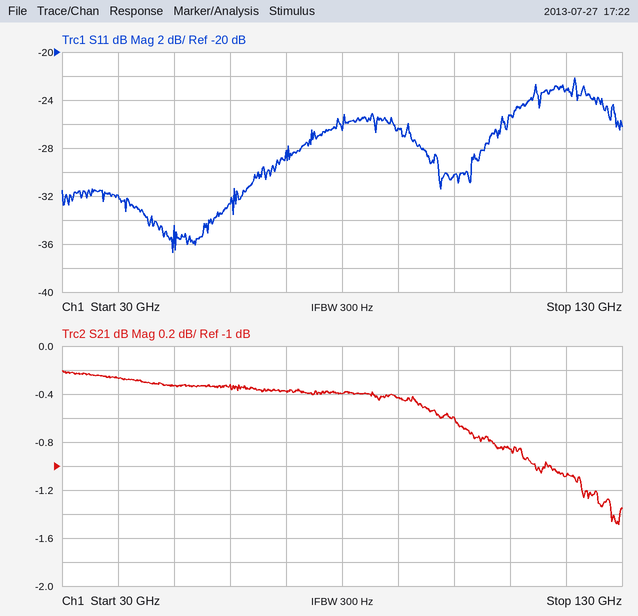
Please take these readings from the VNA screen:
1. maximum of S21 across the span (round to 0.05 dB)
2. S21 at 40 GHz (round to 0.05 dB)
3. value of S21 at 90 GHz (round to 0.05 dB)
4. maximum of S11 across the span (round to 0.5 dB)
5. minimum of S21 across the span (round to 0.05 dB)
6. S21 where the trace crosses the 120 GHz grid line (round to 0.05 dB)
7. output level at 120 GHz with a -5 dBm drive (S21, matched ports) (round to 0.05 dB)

-0.20 dB
-0.25 dB
-0.45 dB
-22.0 dB
-1.50 dB
-1.10 dB
-6.10 dBm
